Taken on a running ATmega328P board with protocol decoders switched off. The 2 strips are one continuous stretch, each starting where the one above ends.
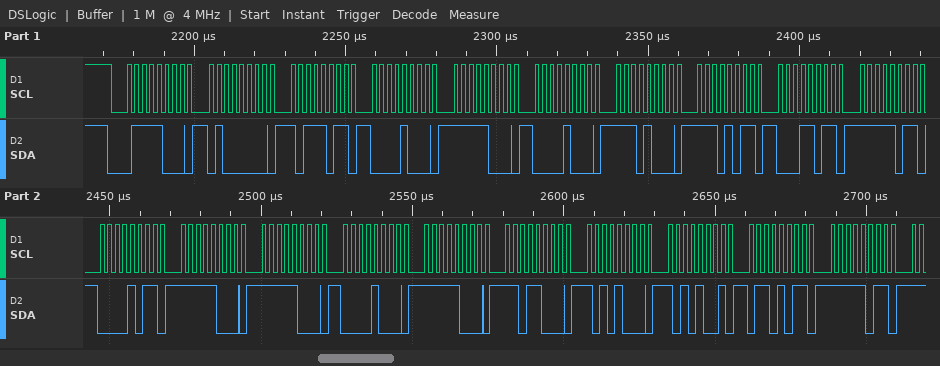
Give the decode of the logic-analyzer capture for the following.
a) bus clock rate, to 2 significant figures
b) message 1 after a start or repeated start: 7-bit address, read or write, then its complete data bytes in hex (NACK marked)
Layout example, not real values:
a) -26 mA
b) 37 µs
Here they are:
a) 400 kHz
b) 0x3C write: 40 BB 08 F8 08 E8 EB 1B FB 0B F8 F8 08 F8 D8 A8 A9 6B FB
